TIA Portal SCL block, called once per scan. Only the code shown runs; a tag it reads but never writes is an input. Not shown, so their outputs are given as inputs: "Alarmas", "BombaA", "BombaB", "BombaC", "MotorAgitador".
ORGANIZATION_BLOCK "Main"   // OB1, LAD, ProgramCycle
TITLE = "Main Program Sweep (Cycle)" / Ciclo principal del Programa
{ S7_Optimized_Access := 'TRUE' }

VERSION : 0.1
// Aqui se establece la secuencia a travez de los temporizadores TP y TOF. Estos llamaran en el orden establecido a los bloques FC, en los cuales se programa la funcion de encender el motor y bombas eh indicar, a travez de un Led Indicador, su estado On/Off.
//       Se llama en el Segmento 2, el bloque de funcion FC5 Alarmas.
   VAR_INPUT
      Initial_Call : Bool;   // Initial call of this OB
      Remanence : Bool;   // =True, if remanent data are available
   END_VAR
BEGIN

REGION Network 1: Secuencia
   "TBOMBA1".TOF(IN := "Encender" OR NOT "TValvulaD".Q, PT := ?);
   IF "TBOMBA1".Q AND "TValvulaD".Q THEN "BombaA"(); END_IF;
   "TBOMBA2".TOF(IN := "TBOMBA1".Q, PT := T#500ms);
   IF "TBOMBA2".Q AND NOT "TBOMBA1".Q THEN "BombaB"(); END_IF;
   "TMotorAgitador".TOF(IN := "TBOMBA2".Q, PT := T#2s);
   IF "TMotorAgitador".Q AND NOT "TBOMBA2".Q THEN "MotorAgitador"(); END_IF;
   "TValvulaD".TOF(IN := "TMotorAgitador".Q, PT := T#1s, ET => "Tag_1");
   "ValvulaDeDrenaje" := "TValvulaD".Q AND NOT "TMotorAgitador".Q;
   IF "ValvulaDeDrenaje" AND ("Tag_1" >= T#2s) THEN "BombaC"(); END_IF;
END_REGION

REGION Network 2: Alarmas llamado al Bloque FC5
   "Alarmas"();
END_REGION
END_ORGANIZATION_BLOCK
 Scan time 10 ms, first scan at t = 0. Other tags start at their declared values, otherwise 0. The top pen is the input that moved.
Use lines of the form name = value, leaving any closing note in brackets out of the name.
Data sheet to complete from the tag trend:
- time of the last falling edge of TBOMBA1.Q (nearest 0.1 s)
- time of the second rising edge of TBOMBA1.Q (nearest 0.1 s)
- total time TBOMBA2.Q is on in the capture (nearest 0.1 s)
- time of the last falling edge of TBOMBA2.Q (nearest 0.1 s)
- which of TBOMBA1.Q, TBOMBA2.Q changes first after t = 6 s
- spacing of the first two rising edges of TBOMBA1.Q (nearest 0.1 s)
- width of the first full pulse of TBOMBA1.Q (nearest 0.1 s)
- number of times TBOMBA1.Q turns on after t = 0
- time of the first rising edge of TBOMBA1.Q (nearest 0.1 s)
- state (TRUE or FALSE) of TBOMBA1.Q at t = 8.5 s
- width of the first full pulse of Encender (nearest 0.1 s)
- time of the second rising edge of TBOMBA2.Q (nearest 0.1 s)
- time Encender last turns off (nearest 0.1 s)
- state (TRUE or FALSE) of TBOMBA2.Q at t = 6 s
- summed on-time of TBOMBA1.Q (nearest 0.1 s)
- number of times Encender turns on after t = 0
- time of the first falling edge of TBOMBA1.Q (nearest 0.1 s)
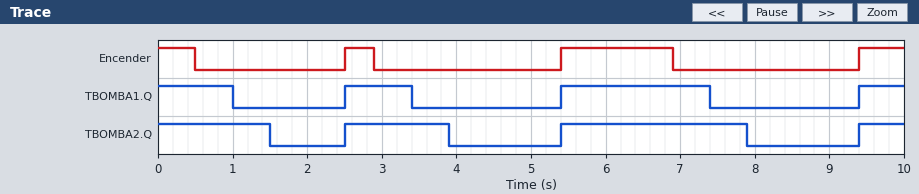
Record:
time of the last falling edge of TBOMBA1.Q = 7.4 s
time of the second rising edge of TBOMBA1.Q = 5.4 s
total time TBOMBA2.Q is on in the capture = 6.0 s
time of the last falling edge of TBOMBA2.Q = 7.9 s
which of TBOMBA1.Q, TBOMBA2.Q changes first after t = 6 s = TBOMBA1.Q
spacing of the first two rising edges of TBOMBA1.Q = 2.9 s
width of the first full pulse of TBOMBA1.Q = 0.9 s
number of times TBOMBA1.Q turns on after t = 0 = 3
time of the first rising edge of TBOMBA1.Q = 2.5 s
state (TRUE or FALSE) of TBOMBA1.Q at t = 8.5 s = FALSE
width of the first full pulse of Encender = 0.4 s
time of the second rising edge of TBOMBA2.Q = 5.4 s
time Encender last turns off = 6.9 s
state (TRUE or FALSE) of TBOMBA2.Q at t = 6 s = TRUE
summed on-time of TBOMBA1.Q = 4.5 s
number of times Encender turns on after t = 0 = 3
time of the first falling edge of TBOMBA1.Q = 1.0 s
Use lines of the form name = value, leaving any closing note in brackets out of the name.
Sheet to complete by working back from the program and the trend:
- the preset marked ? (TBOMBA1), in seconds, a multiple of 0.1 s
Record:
the preset marked ? (TBOMBA1), in seconds, a multiple of 0.1 s = 0.5 s
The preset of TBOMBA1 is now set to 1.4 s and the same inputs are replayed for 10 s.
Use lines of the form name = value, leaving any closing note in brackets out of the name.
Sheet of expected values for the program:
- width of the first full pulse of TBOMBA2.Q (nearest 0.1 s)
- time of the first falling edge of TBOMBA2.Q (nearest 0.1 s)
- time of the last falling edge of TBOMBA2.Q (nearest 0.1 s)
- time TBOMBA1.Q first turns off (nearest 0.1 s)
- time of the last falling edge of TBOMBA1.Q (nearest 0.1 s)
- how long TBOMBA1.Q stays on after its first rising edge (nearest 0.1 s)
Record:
width of the first full pulse of TBOMBA2.Q = 2.3 s
time of the first falling edge of TBOMBA2.Q = 2.4 s
time of the last falling edge of TBOMBA2.Q = 8.8 s
time TBOMBA1.Q first turns off = 1.9 s
time of the last falling edge of TBOMBA1.Q = 8.3 s
how long TBOMBA1.Q stays on after its first rising edge = 1.8 s
